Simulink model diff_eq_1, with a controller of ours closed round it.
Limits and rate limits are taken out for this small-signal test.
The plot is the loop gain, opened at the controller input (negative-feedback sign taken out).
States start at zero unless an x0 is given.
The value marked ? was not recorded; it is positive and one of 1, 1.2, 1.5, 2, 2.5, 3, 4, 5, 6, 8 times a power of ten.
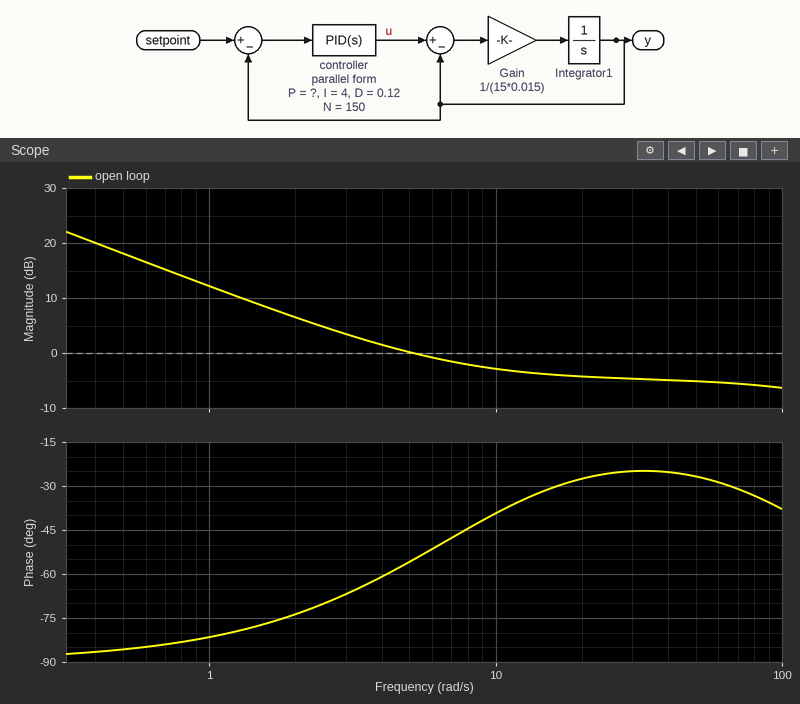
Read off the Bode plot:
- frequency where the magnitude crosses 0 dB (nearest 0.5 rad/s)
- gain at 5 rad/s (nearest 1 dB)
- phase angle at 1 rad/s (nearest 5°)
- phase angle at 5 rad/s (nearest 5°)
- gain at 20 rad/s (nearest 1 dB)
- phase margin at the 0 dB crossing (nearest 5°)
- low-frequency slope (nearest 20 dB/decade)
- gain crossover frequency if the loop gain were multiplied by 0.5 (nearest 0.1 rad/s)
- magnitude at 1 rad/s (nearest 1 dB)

5.0 rad/s
0 dB
-80°
-55°
-4 dB
125°
-20 dB/decade
2.1 rad/s
12 dB
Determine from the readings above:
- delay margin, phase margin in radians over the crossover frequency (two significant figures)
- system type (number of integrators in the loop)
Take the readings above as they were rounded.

0.44 s
1
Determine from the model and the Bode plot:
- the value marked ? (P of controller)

1.5
